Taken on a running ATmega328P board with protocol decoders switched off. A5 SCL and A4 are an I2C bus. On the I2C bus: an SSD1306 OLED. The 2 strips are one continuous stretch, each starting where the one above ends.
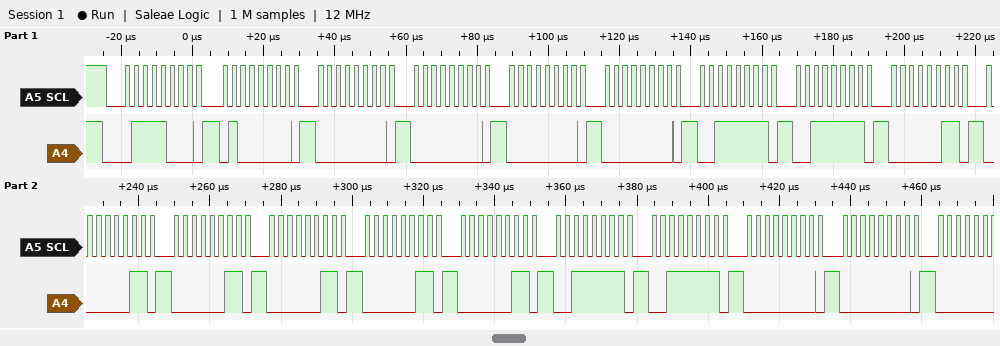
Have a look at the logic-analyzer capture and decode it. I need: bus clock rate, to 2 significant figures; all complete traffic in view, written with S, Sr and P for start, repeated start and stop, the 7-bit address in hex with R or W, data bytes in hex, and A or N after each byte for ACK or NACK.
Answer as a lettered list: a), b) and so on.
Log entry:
a) 400 kHz
b) S 3CW A 40 A 00 A 00 A 00 A 00 A 3F A 3F A 03 A 03 A 03 A 03 A 03 A 03 A 3F A 3F A 00 A 00 A
